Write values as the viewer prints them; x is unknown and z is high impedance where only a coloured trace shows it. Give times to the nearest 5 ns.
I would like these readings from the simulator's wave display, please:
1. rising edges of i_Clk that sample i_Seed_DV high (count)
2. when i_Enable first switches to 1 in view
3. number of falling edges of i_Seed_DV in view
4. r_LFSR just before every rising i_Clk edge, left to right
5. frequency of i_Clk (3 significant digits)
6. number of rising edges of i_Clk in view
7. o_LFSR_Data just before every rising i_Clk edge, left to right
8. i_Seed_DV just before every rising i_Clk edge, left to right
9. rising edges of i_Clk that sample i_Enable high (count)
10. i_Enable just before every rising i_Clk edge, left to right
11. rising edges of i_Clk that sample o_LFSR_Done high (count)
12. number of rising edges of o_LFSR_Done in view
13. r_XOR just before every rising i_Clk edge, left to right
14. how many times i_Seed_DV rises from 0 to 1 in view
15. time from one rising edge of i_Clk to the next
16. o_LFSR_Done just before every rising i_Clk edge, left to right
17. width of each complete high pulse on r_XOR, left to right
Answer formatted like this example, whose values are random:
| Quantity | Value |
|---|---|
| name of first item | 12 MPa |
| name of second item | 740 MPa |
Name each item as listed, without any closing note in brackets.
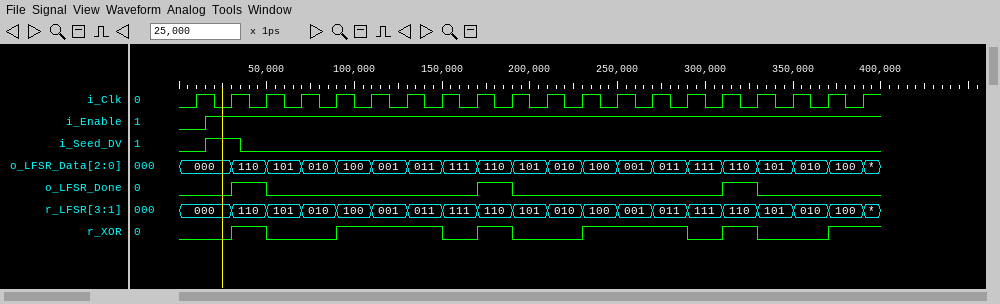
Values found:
| Quantity | Value |
|---|---|
| rising edges of i_Clk that sample i_Seed_DV high | 1 |
| when i_Enable first switches to 1 in view | 15 ns |
| number of falling edges of i_Seed_DV in view | 1 |
| r_LFSR just before every rising i_Clk edge, left to right | 000, 000, 110, 101, 010, 100, 001, 011, 111, 110, 101, 010, 100, 001, 011, 111, 110, 101, 010, 100 |
| frequency of i_Clk | 50.0 MHz |
| number of rising edges of i_Clk in view | 20 |
| o_LFSR_Data just before every rising i_Clk edge, left to right | 000, 000, 110, 101, 010, 100, 001, 011, 111, 110, 101, 010, 100, 001, 011, 111, 110, 101, 010, 100 |
| i_Seed_DV just before every rising i_Clk edge, left to right | 0 1 0 0 0 0 0 0 0 0 0 0 0 0 0 0 0 0 0 0 |
| rising edges of i_Clk that sample i_Enable high | 19 |
| i_Enable just before every rising i_Clk edge, left to right | 0 1 1 1 1 1 1 1 1 1 1 1 1 1 1 1 1 1 1 1 |
| rising edges of i_Clk that sample o_LFSR_Done high | 3 |
| number of rising edges of o_LFSR_Done in view | 3 |
| r_XOR just before every rising i_Clk edge, left to right | 0 0 1 0 0 1 1 1 0 1 0 0 1 1 1 0 1 0 0 1 |
| how many times i_Seed_DV rises from 0 to 1 in view | 1 |
| time from one rising edge of i_Clk to the next | 20 ns |
| o_LFSR_Done just before every rising i_Clk edge, left to right | 0 0 1 0 0 0 0 0 0 1 0 0 0 0 0 0 1 0 0 0 |
| width of each complete high pulse on r_XOR, left to right | 20 ns, 60 ns, 20 ns, 60 ns, 20 ns |
